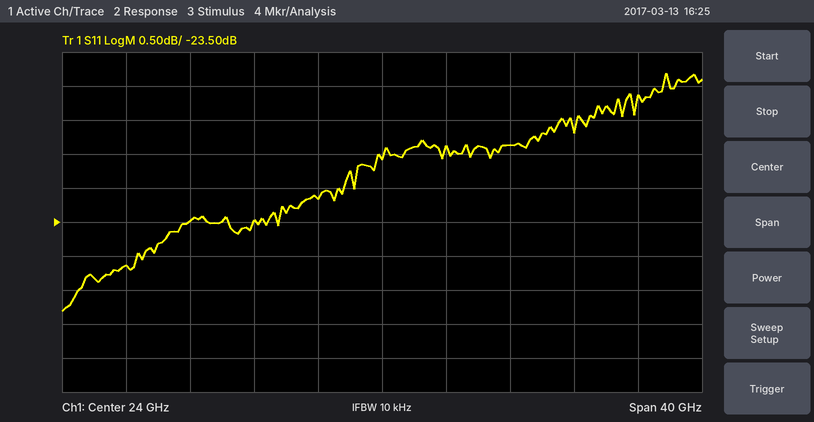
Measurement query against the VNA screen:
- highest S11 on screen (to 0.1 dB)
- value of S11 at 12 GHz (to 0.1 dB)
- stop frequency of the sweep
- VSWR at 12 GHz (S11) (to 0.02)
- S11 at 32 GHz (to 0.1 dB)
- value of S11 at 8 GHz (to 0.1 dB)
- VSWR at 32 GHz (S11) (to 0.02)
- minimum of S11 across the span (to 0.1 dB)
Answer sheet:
-21.3 dB
-23.5 dB
44 GHz
1.14
-22.4 dB
-24.1 dB
1.16
-24.8 dB
